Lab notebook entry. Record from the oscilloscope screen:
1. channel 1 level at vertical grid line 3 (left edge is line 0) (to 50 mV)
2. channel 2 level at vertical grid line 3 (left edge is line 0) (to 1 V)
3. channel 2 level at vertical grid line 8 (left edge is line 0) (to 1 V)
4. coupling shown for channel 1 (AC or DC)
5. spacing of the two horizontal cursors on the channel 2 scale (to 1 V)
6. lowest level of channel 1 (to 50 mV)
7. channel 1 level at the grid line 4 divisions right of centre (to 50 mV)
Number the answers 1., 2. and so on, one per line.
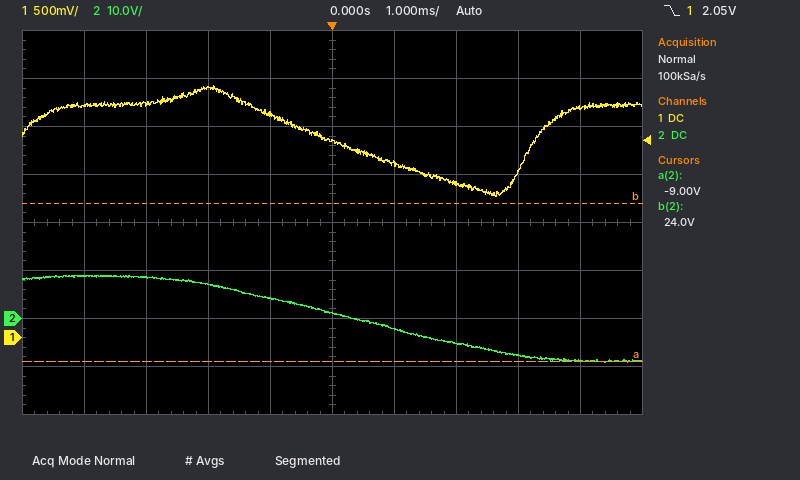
1. 2.60 V
2. 7 V
3. -8 V
4. DC
5. 33 V
6. 1.45 V
7. 2.40 V
